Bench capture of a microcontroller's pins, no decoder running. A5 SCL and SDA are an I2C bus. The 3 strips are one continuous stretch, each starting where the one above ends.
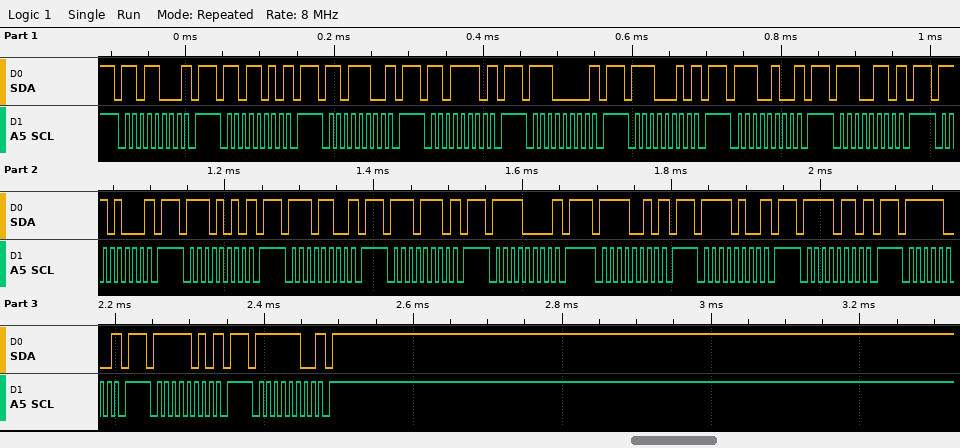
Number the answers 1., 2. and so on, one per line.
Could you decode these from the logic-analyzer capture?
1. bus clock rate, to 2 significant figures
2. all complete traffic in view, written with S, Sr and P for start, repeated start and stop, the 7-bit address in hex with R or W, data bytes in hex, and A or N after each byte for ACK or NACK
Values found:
1. 100 kHz
2. S 6CW N P S 6DW N P S 6EW N P S 6FW N P S 70W N P S 71W N P S 72W N P S 73W N P S 74W N P S 75W N P S 76W N P S 77W N P S 78W N P S 79W N P S 7AW N P S 7BW N P S 7CW N P S 7DW N P S 7EW N P
